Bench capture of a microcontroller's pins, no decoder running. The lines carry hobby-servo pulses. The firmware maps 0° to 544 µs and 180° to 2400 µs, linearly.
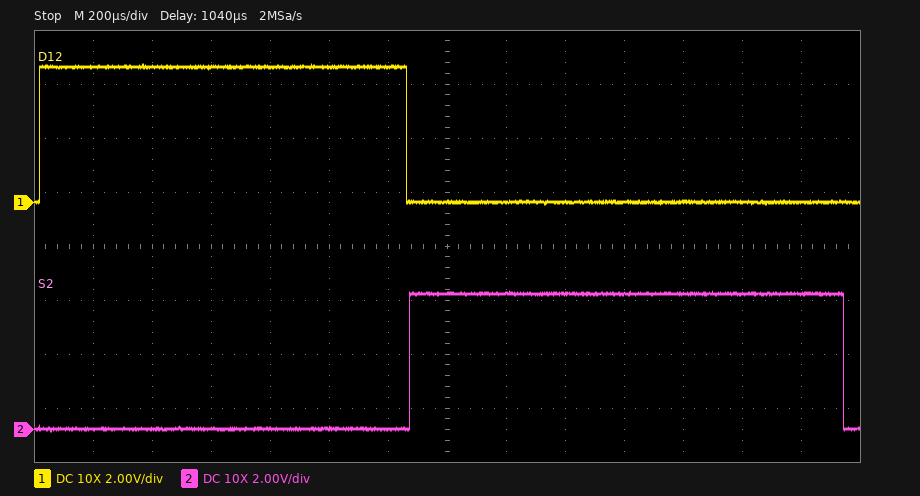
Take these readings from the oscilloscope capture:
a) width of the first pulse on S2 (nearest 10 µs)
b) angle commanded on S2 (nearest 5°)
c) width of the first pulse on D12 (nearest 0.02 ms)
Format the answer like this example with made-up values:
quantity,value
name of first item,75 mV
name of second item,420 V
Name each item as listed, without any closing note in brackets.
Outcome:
quantity,value
width of the first pulse on S2,1470 µs
angle commanded on S2,90°
width of the first pulse on D12,1.24 ms
